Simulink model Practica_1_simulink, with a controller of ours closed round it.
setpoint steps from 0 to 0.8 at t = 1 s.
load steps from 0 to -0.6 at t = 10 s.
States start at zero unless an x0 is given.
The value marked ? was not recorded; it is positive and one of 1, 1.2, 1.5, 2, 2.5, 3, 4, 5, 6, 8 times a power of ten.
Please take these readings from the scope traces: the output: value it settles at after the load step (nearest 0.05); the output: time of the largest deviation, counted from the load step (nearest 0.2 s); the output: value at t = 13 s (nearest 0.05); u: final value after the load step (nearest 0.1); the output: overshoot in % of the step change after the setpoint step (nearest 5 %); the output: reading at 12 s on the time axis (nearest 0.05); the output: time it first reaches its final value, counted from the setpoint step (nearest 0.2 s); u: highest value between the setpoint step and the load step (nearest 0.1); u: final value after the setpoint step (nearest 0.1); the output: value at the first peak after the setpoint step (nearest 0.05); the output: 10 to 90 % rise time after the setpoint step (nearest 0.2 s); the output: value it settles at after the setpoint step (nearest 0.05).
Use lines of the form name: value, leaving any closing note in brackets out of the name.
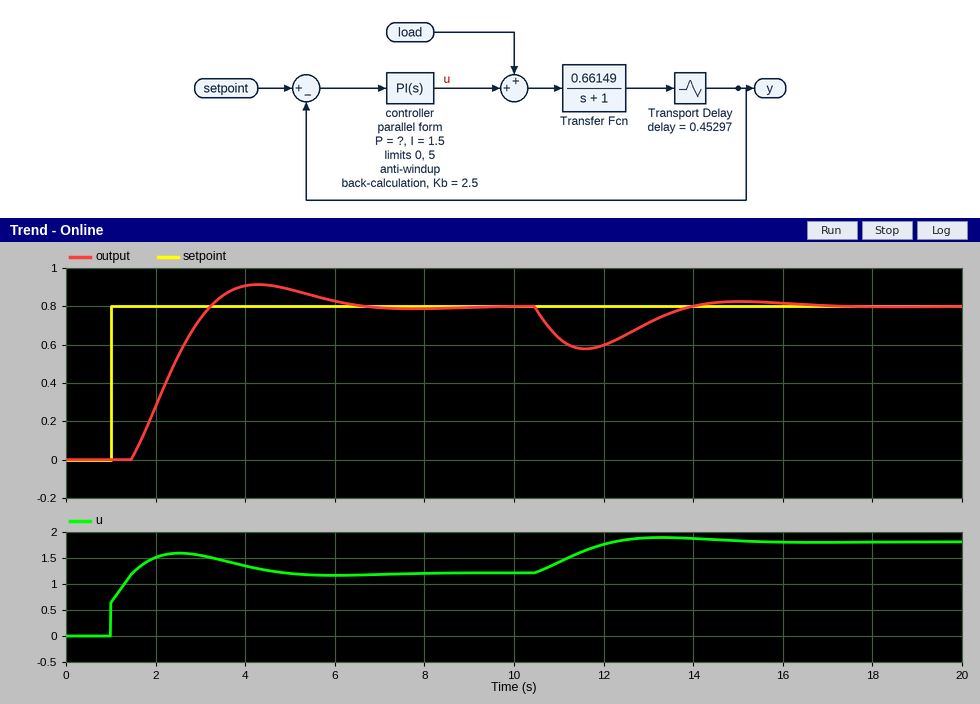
the output: value it settles at after the load step: 0.80
the output: time of the largest deviation, counted from the load step: 1.6 s
the output: value at t = 13 s: 0.70
u: final value after the load step: 1.8
the output: overshoot in % of the step change after the setpoint step: 15 %
the output: reading at 12 s on the time axis: 0.60
the output: time it first reaches its final value, counted from the setpoint step: 2.2 s
u: highest value between the setpoint step and the load step: 1.6
u: final value after the setpoint step: 1.2
the output: value at the first peak after the setpoint step: 0.90
the output: 10 to 90 % rise time after the setpoint step: 1.4 s
the output: value it settles at after the setpoint step: 0.80
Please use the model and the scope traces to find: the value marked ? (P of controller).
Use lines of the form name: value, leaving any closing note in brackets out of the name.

the value marked ?: 0.8
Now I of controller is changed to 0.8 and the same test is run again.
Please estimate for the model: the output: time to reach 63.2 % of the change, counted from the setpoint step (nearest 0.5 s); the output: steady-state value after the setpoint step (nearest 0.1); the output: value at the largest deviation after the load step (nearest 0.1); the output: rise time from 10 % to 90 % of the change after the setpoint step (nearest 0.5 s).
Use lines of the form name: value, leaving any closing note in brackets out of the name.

the output: time to reach 63.2 % of the change, counted from the setpoint step: 2.0 s
the output: steady-state value after the setpoint step: 0.8
the output: value at the largest deviation after the load step: 0.6
the output: rise time from 10 % to 90 % of the change after the setpoint step: 3.0 s
